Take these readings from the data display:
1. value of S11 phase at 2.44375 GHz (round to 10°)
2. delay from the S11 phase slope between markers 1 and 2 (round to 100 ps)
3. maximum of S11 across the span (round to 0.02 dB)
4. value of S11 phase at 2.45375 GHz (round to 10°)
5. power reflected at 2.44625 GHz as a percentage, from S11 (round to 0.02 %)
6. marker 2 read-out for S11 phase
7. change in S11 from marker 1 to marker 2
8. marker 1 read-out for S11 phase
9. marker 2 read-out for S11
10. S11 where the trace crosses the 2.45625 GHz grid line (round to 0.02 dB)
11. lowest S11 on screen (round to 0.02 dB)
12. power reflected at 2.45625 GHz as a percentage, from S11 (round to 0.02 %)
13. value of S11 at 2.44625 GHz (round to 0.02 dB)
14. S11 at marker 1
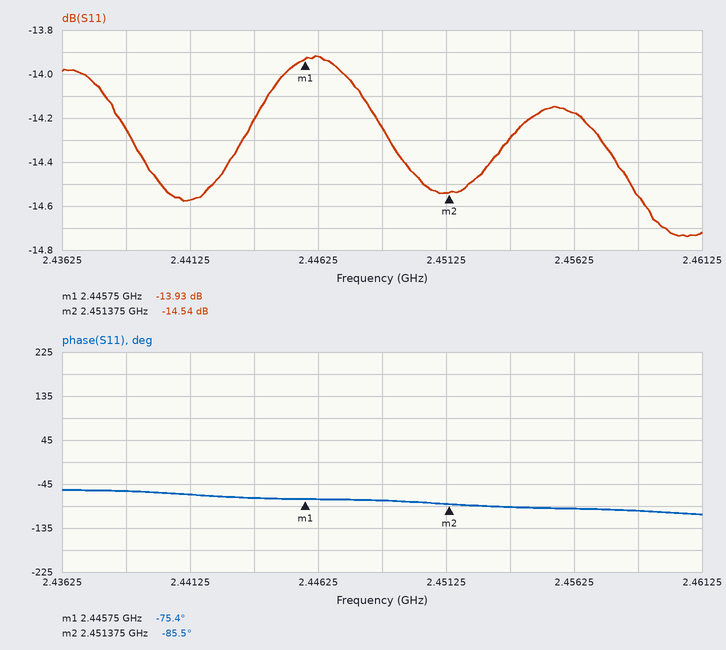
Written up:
-70°
5.0 ns
-13.92 dB
-90°
4.06 %
-85.5°
-0.61 dB
-75.4°
-14.54 dB
-14.18 dB
-14.74 dB
3.82 %
-13.92 dB
-13.93 dB
